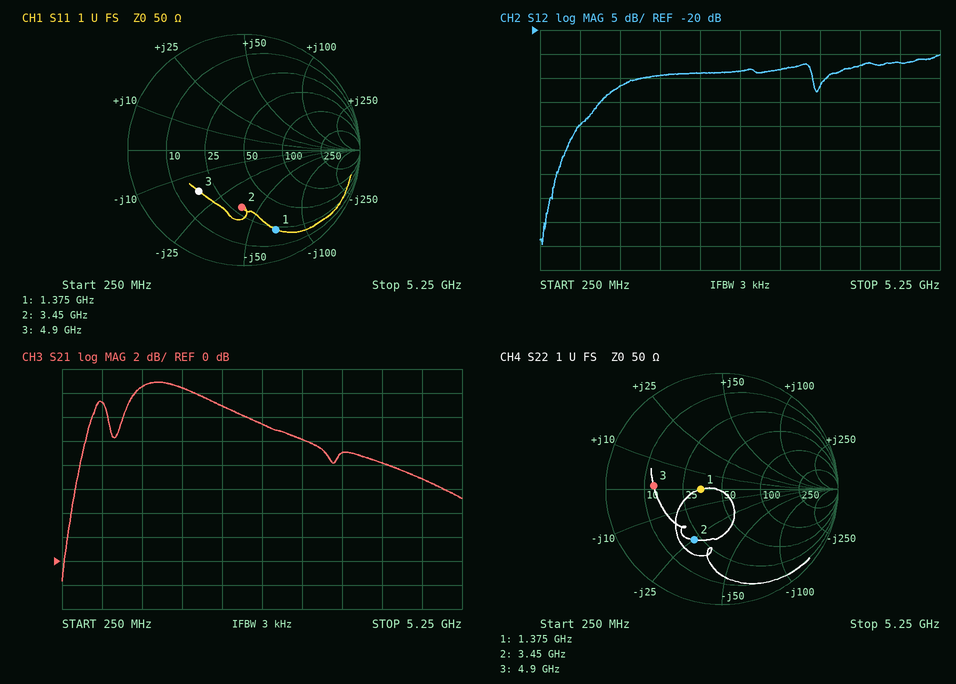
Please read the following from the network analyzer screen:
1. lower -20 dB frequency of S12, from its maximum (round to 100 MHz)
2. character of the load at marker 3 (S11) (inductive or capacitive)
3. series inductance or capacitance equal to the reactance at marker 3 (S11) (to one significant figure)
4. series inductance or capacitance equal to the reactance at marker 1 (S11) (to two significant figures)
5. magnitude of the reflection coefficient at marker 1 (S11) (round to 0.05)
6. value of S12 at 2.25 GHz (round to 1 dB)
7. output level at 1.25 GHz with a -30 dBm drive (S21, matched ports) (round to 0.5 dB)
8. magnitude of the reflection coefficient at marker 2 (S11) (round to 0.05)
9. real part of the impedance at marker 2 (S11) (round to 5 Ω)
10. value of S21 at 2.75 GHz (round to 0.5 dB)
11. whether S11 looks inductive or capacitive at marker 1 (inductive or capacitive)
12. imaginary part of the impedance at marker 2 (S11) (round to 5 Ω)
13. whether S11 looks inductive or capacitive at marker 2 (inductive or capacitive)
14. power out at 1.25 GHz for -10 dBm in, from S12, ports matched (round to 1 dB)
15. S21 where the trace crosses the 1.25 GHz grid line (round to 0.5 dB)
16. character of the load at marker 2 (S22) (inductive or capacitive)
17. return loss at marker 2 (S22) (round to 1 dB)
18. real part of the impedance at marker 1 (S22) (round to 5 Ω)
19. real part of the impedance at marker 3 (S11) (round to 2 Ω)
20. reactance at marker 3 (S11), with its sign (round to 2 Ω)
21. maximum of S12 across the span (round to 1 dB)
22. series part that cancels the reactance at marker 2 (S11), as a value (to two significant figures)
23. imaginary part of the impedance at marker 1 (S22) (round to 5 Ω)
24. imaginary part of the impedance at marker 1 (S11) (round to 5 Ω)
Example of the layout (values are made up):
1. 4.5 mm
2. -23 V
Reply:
1. 600 MHz
2. capacitive
3. 2 pF
4. 1.7 pF
5. 0.75
6. -29 dB
7. -15.5 dBm
8. 0.50
9. 30 Ω
10. 11.5 dB
11. capacitive
12. -40 Ω
13. capacitive
14. -42 dBm
15. 14.5 dB
16. capacitive
17. 6 dB
18. 35 Ω
19. 18 Ω
20. -18 Ω
21. -25 dB
22. 1.8 nH
23. 0 Ω
24. -70 Ω
